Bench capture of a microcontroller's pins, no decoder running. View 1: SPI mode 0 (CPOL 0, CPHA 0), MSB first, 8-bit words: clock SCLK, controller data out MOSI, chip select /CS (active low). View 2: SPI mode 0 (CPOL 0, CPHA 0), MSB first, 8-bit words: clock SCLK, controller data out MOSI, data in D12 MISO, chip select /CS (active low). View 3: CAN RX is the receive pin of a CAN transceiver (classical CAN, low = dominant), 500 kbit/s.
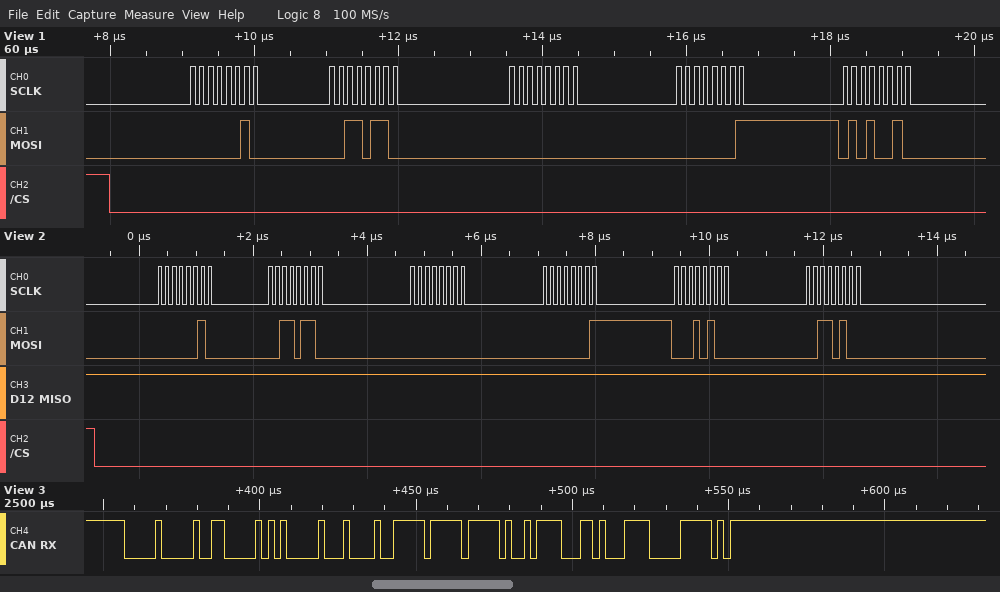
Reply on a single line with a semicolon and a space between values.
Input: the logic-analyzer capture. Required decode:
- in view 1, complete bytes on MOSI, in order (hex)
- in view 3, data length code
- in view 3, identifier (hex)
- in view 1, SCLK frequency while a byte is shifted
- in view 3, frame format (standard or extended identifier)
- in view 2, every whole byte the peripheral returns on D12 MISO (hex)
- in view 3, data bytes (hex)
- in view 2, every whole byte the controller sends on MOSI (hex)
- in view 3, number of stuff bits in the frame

02 36 00 01 52; 4; 0x00000A01; 8 MHz; extended; FF FF FF FF FF FF; FF FF 2F 1A; 02 36 00 01 14 34; 9
